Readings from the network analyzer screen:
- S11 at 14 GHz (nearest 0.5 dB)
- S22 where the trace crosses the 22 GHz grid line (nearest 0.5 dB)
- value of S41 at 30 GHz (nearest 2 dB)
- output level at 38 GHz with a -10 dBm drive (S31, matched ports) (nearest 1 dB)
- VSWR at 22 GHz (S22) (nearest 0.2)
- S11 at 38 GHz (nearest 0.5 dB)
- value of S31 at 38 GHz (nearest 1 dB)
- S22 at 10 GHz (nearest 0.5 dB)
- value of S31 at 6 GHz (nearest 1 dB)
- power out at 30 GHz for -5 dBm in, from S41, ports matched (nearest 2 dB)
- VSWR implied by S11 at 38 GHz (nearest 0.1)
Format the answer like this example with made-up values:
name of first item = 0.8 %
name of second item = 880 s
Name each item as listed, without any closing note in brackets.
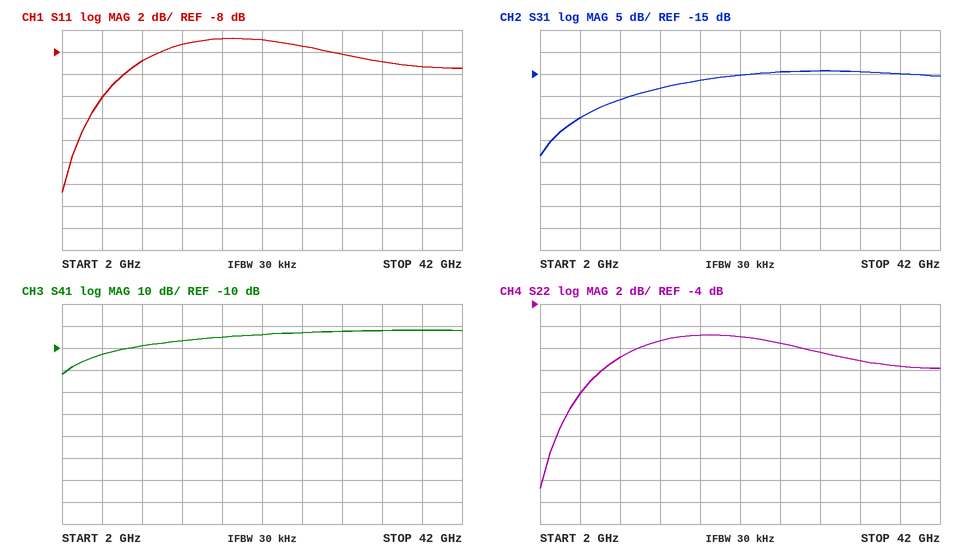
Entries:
S11 at 14 GHz = -7.5 dB
S22 where the trace crosses the 22 GHz grid line = -7.0 dB
value of S41 at 30 GHz = -2 dB
output level at 38 GHz with a -10 dBm drive (S31, matched ports) = -25 dBm
VSWR at 22 GHz (S22) = 2.6
S11 at 38 GHz = -9.5 dB
value of S31 at 38 GHz = -15 dB
S22 at 10 GHz = -9.0 dB
value of S31 at 6 GHz = -25 dB
power out at 30 GHz for -5 dBm in, from S41, ports matched = -8 dBm
VSWR implied by S11 at 38 GHz = 2.0
